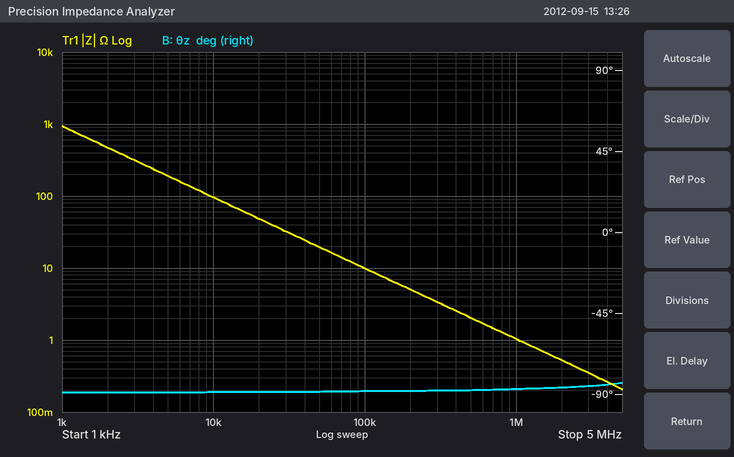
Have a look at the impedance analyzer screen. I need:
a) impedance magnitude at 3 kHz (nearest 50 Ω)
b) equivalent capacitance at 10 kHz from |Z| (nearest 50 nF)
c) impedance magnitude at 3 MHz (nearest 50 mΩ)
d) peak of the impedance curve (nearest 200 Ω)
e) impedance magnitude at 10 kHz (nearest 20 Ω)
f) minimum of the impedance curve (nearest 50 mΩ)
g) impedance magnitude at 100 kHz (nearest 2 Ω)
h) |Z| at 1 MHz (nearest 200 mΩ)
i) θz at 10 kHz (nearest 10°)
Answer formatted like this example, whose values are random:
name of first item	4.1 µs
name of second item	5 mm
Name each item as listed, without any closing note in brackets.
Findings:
impedance magnitude at 3 kHz	300 Ω
equivalent capacitance at 10 kHz from |Z|	150 nF
impedance magnitude at 3 MHz	350 mΩ
peak of the impedance curve	1.0 kΩ
impedance magnitude at 10 kHz	100 Ω
minimum of the impedance curve	200 mΩ
impedance magnitude at 100 kHz	10 Ω
|Z| at 1 MHz	1.0 Ω
θz at 10 kHz	-90°
